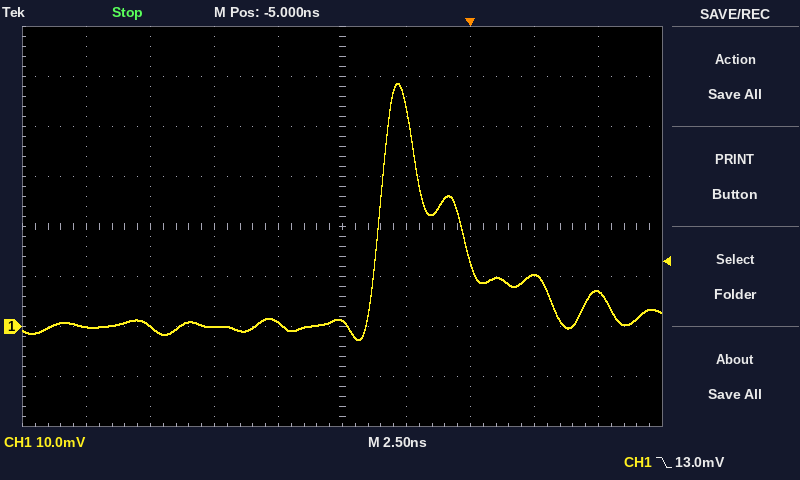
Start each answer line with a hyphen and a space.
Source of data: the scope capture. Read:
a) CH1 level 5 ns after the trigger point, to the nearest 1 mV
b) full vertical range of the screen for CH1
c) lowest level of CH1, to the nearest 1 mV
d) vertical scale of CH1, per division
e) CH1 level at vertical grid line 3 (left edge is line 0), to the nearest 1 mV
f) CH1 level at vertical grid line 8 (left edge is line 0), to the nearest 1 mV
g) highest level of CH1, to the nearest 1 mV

- 7 mV
- 80 mV
- -3 mV
- 10 mV
- 0 mV
- 10 mV
- 49 mV
